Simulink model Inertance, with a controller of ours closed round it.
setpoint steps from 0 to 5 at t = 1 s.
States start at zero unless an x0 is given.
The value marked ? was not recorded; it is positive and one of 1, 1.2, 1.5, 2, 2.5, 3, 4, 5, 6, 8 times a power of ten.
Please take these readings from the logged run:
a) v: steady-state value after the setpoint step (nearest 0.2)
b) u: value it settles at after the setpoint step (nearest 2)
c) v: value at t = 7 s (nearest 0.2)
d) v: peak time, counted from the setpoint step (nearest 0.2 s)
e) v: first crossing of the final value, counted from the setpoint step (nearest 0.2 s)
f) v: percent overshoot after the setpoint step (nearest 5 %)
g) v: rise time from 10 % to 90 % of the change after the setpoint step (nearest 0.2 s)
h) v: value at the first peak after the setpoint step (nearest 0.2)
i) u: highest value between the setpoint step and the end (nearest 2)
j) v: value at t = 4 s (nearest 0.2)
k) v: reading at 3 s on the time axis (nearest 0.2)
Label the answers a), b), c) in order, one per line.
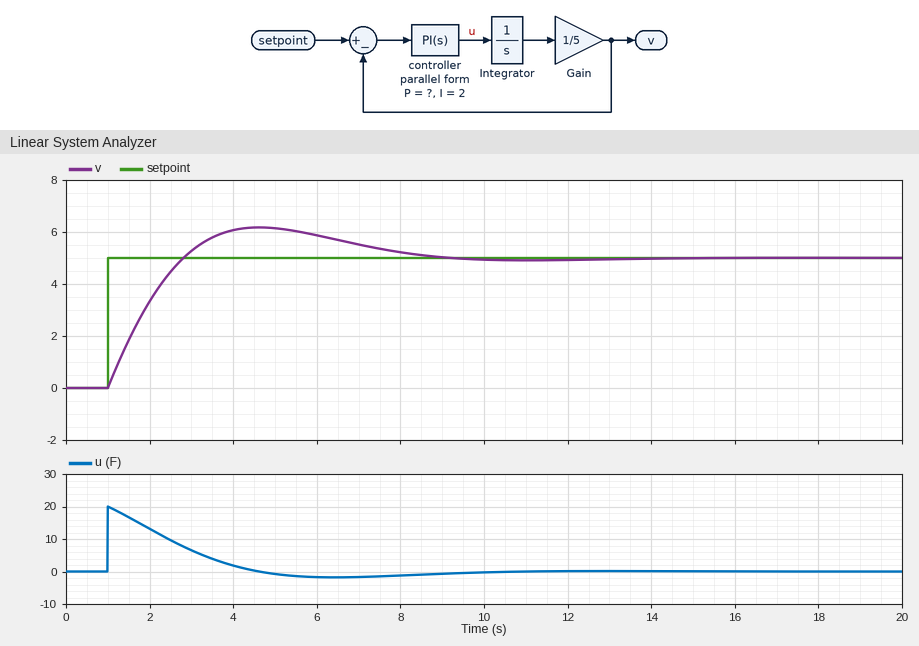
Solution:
a) 5.0
b) 0
c) 5.6
d) 3.6 s
e) 1.8 s
f) 25 %
g) 1.4 s
h) 6.2
i) 20
j) 6.0
k) 5.2
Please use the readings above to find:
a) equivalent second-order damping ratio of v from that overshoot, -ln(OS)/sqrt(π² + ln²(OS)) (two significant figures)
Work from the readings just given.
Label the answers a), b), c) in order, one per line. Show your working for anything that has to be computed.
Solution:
a) ln(0.25) = -1.386; 1.386 / sqrt(9.870 + 1.922) = 0.40
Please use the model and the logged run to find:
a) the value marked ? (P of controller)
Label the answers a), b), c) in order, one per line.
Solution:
a) 4
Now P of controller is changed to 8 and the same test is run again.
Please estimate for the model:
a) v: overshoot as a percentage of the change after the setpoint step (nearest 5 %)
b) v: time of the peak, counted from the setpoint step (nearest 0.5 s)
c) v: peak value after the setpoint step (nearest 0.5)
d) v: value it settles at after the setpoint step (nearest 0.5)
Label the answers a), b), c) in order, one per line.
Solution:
a) 10 %
b) 3.0 s
c) 5.5
d) 5.0
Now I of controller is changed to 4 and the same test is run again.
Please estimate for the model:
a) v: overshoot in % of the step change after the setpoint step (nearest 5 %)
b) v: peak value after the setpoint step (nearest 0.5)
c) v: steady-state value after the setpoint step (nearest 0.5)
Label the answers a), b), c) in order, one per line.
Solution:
a) 35 %
b) 6.5
c) 5.0
